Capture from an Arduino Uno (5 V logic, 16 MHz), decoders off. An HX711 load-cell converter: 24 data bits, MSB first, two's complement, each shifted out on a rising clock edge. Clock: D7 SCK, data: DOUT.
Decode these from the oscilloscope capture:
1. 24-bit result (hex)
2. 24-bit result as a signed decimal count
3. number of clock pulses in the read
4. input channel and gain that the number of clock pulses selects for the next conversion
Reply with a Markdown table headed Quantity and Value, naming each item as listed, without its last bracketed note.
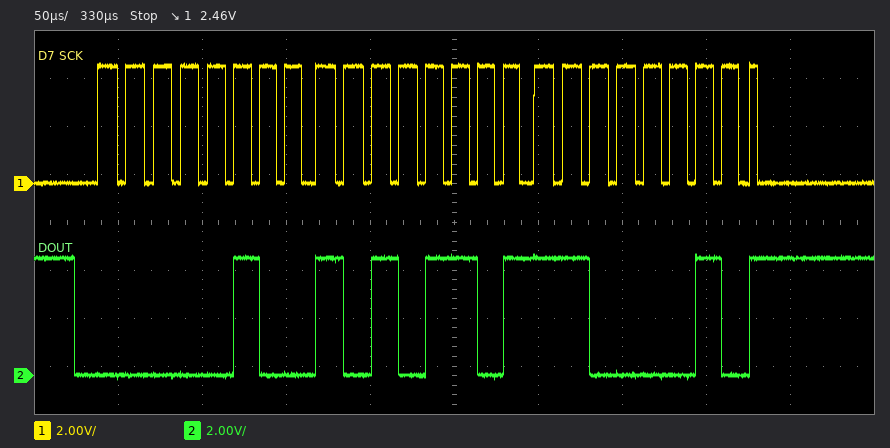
| Quantity | Value |
|---|---|
| 24-bit result | 0x04ADC2 |
| 24-bit result as a signed decimal count | 306626 |
| number of clock pulses in the read | 25 |
| input channel and gain that the number of clock pulses selects for the next conversion | channel A, gain 128 |
